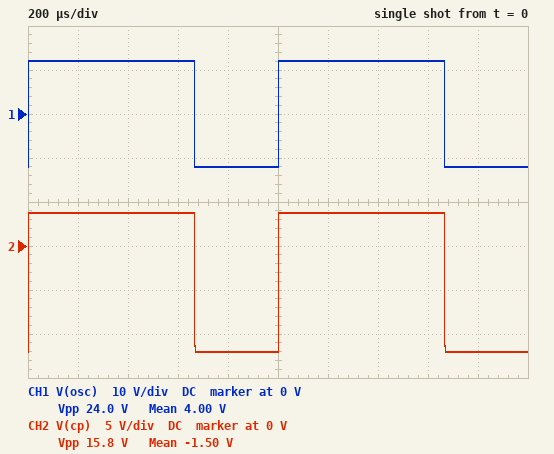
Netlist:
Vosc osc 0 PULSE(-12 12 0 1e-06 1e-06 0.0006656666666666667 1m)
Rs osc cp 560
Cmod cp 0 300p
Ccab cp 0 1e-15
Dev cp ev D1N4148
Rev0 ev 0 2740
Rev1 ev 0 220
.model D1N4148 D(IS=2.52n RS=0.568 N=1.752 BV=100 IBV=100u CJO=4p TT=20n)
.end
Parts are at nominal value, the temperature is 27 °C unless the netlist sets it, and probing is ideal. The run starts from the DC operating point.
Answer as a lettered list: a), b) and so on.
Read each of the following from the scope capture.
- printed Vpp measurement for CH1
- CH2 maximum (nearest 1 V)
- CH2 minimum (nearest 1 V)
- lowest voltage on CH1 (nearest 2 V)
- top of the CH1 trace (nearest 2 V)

a) 24.0 V
b) 4 V
c) -12 V
d) -12 V
e) 12 V
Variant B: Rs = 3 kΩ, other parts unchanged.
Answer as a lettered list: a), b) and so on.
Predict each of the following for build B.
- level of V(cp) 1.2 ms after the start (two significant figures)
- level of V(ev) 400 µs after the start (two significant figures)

a) 1.4 V
b) 720 mV
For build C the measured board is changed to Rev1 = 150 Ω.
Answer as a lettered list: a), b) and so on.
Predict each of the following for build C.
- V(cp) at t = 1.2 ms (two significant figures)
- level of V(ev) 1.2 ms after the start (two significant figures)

a) 3.0 V
b) 2.3 V
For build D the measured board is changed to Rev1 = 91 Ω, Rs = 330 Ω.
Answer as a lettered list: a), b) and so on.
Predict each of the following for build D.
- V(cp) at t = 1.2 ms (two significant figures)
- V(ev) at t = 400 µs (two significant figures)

a) 3.1 V
b) 2.4 V
